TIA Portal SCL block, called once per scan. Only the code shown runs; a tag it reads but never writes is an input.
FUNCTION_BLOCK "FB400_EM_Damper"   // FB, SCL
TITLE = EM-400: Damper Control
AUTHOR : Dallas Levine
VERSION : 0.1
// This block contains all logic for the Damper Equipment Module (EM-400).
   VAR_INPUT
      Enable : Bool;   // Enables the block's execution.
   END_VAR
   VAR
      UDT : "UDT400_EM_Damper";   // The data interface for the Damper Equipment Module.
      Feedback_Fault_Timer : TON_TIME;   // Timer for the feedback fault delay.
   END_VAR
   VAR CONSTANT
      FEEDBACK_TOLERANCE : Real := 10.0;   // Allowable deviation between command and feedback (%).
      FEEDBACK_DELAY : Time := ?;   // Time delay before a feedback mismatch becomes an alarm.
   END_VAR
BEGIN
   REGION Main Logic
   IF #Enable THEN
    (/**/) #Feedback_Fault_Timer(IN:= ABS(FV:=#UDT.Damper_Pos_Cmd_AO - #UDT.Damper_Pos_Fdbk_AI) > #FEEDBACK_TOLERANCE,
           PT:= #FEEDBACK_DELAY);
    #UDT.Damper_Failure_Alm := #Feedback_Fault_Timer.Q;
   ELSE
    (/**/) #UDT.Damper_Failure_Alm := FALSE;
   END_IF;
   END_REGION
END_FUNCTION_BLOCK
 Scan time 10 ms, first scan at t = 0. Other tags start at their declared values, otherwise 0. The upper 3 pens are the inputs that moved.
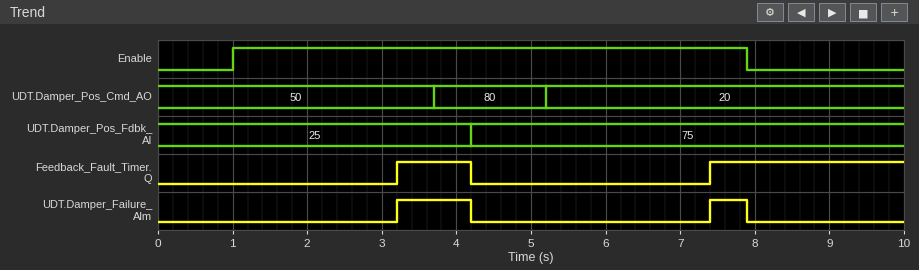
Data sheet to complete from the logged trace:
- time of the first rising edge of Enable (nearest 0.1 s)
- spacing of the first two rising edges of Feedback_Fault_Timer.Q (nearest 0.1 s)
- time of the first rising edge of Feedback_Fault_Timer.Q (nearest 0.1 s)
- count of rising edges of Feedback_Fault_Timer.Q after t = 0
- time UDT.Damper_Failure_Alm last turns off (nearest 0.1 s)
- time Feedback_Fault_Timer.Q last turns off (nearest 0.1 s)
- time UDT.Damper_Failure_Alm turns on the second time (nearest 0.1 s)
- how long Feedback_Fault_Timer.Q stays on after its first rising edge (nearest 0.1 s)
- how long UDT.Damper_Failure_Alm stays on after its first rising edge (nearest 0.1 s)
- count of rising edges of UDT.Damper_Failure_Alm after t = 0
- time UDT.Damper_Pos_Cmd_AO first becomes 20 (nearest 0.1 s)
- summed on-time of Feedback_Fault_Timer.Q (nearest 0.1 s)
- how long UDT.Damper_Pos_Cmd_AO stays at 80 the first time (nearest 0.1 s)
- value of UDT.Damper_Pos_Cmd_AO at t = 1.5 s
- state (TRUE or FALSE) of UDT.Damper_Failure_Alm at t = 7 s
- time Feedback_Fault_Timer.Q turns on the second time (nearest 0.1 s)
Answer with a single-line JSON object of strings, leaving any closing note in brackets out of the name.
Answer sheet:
{"time of the first rising edge of Enable": "1.0 s", "spacing of the first two rising edges of Feedback_Fault_Timer.Q": "4.2 s", "time of the first rising edge of Feedback_Fault_Timer.Q": "3.2 s", "count of rising edges of Feedback_Fault_Timer.Q after t = 0": "2", "time UDT.Damper_Failure_Alm last turns off": "7.9 s", "time Feedback_Fault_Timer.Q last turns off": "4.2 s", "time UDT.Damper_Failure_Alm turns on the second time": "7.4 s", "how long Feedback_Fault_Timer.Q stays on after its first rising edge": "1.0 s", "how long UDT.Damper_Failure_Alm stays on after its first rising edge": "1.0 s", "count of rising edges of UDT.Damper_Failure_Alm after t = 0": "2", "time UDT.Damper_Pos_Cmd_AO first becomes 20": "5.2 s", "summed on-time of Feedback_Fault_Timer.Q": "3.6 s", "how long UDT.Damper_Pos_Cmd_AO stays at 80 the first time": "1.5 s", "value of UDT.Damper_Pos_Cmd_AO at t = 1.5 s": "50", "state (TRUE or FALSE) of UDT.Damper_Failure_Alm at t = 7 s": "FALSE", "time Feedback_Fault_Timer.Q turns on the second time": "7.4 s"}
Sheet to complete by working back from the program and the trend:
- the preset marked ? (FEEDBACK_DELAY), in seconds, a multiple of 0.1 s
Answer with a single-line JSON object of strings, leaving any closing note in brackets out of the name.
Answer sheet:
{"the preset marked ? (FEEDBACK_DELAY), in seconds, a multiple of 0.1 s": "2.2 s"}
